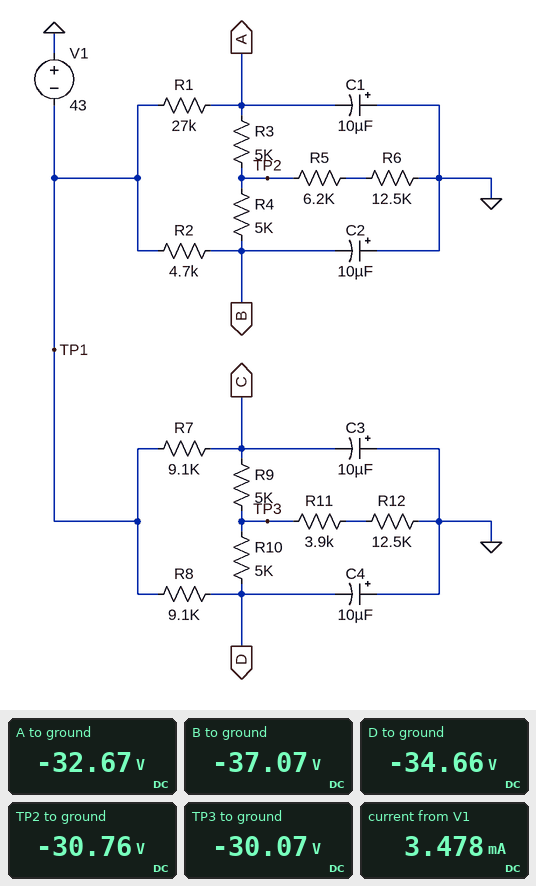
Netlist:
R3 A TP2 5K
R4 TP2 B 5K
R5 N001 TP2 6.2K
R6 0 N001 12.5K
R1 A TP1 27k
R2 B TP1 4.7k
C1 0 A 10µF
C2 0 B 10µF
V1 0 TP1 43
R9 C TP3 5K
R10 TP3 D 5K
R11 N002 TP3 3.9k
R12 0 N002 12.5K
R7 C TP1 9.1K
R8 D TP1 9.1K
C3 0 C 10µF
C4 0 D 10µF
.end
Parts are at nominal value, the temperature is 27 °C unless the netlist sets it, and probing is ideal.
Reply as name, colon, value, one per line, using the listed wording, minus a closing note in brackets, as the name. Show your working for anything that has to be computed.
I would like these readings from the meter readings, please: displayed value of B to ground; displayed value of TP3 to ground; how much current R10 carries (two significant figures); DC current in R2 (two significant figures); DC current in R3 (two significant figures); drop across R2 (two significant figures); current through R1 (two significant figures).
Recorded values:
displayed value of B to ground: -37.07 V
displayed value of TP3 to ground: -30.07 V
how much current R10 carries: (-30.07 V - (-34.66 V)) / 5 kΩ = 920 µA
DC current in R2: (-37.07 V - (-43 V)) / 4.7 kΩ = 1.3 mA
DC current in R3: (-30.76 V - (-32.67 V)) / 5 kΩ = 380 µA
drop across R2: -37.07 V - (-43 V) = 5.9 V
current through R1: (-32.67 V - (-43 V)) / 27 kΩ = 380 µA
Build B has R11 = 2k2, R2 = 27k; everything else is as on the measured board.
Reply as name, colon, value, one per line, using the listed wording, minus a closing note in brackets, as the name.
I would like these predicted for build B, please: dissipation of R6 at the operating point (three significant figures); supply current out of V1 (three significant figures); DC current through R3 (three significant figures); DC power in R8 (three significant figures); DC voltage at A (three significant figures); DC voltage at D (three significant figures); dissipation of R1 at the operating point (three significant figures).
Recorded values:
dissipation of R6 at the operating point: 19.2 mW
supply current out of V1: 3.22 mA
DC current through R3: 620 µA
DC power in R8: 8.89 mW
DC voltage at A: -26.3 V
DC voltage at D: -34.0 V
dissipation of R1 at the operating point: 10.4 mW
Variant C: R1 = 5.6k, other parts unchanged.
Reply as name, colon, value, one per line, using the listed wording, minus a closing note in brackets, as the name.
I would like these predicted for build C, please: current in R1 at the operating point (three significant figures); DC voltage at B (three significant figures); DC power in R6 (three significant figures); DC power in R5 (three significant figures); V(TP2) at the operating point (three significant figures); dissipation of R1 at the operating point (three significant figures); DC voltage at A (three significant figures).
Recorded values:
current in R1 at the operating point: 865 µA
DC voltage at B: -38.6 V
DC power in R6: 40.9 mW
DC power in R5: 20.3 mW
V(TP2) at the operating point: -33.8 V
dissipation of R1 at the operating point: 4.19 mW
DC voltage at A: -38.2 V
